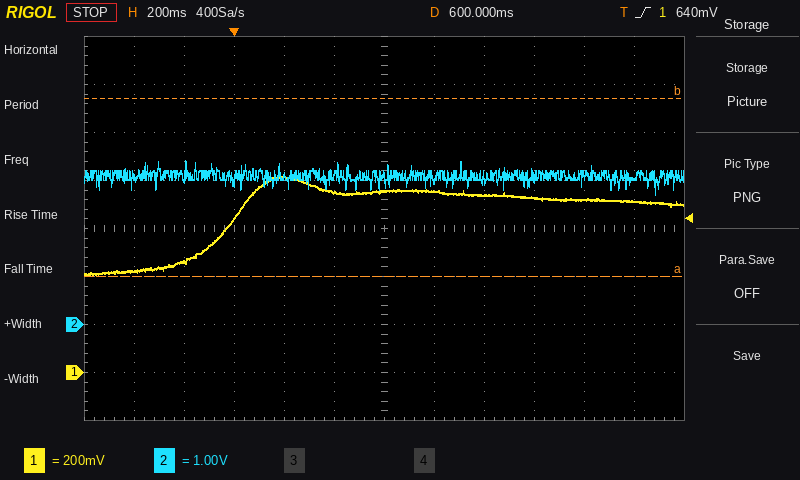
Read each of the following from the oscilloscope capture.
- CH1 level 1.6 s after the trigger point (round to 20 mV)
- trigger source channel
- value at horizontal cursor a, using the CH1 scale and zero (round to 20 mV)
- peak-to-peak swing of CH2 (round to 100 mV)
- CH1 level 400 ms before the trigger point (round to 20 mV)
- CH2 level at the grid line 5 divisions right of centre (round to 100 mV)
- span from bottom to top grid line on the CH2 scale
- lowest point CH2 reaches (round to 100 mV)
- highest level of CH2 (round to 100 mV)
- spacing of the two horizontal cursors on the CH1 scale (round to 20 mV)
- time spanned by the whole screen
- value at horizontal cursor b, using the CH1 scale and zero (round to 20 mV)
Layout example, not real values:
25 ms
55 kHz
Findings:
720 mV
CH1
400 mV
700 mV
420 mV
3.1 V
8 V
2.7 V
3.4 V
740 mV
2.4 s
1.14 V
